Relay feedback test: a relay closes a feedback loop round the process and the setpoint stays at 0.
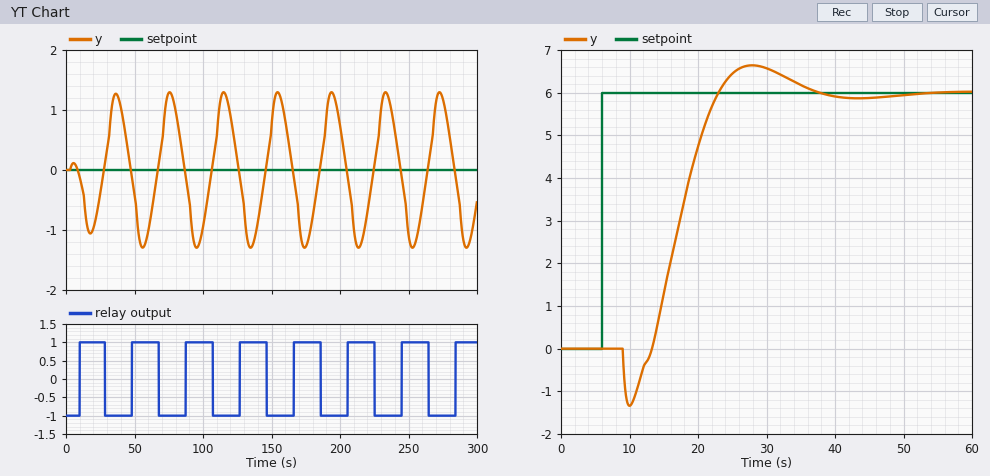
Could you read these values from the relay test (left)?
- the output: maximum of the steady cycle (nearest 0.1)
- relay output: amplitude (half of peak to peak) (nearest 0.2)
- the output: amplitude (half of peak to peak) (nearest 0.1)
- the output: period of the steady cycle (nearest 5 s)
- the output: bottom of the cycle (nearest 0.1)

1.3
1.0
1.3
40 s
-1.3
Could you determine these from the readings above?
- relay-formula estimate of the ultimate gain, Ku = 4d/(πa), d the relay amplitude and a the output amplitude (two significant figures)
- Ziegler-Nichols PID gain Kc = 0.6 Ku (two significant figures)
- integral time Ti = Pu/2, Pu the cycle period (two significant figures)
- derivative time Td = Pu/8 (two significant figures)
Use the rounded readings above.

0.98
0.59
20 s
5.0 s
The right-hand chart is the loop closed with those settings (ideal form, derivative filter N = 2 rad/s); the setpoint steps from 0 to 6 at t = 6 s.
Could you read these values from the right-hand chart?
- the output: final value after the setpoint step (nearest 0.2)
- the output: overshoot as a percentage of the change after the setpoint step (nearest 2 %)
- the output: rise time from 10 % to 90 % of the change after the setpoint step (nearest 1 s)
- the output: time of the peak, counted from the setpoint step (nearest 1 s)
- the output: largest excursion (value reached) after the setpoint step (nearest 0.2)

6.0
10 %
7 s
22 s
6.6
